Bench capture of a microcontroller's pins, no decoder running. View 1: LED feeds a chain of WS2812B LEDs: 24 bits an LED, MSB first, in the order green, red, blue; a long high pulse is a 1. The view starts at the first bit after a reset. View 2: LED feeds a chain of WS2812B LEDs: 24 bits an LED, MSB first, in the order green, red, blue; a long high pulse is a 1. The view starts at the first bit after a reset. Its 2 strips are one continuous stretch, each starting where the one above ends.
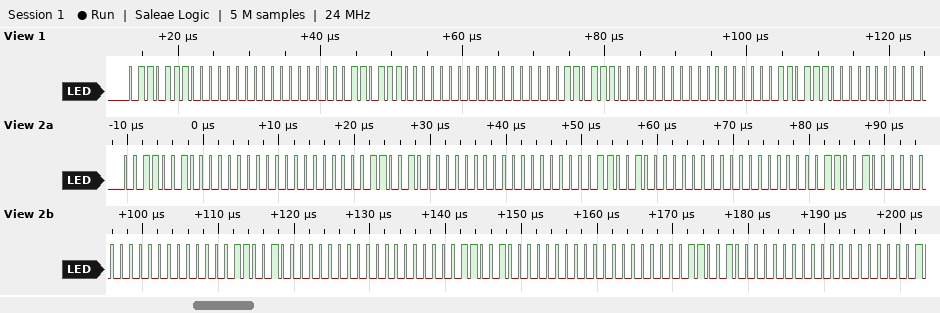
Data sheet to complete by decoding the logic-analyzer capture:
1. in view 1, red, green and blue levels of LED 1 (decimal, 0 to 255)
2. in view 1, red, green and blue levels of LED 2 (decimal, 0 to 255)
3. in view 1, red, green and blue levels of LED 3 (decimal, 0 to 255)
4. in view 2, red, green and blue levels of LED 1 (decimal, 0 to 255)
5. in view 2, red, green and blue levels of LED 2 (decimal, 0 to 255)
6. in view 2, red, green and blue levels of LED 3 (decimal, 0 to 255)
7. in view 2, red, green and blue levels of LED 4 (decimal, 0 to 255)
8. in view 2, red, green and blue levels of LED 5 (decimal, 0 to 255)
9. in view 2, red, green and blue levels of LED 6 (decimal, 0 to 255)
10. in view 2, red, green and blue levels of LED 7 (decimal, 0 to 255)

0, 110, 0
0, 110, 0
0, 110, 0
0, 50, 0
0, 50, 0
0, 50, 0
0, 50, 0
0, 50, 0
0, 50, 0
0, 50, 0
